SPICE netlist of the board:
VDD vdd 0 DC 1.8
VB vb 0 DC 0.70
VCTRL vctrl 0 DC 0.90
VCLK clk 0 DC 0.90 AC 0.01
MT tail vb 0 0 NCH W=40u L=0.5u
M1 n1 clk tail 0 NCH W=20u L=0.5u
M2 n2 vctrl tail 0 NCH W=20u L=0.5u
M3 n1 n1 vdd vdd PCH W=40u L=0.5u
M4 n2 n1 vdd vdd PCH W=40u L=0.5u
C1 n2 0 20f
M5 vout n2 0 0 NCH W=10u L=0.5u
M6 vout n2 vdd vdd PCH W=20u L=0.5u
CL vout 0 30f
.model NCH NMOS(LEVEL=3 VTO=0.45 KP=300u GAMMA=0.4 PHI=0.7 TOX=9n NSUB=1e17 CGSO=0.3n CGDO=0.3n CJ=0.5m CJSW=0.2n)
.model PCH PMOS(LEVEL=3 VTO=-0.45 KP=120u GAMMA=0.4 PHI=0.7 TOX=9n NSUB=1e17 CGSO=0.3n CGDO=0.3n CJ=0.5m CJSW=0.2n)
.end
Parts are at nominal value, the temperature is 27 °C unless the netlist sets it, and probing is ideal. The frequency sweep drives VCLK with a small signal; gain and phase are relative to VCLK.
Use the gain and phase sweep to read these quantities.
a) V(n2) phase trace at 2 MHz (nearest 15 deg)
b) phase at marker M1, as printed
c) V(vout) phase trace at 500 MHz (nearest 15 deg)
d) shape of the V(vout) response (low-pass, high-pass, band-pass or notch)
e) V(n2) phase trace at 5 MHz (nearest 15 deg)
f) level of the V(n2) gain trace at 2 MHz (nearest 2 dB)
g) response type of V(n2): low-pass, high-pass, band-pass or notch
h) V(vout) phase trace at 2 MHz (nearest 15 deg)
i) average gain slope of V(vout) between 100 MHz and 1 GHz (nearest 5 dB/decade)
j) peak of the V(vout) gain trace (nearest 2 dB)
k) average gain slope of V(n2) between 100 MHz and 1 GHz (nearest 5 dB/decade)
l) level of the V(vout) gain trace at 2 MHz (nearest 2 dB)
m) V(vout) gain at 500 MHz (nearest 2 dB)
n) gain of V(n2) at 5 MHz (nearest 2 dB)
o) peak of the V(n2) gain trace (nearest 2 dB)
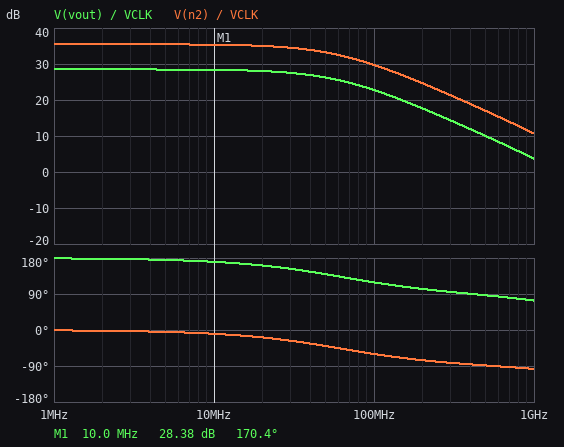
0 deg
170.4 deg
90 deg
low-pass
0 deg
36 dB
low-pass
180 deg
-20 dB/decade
28 dB
-20 dB/decade
28 dB
10 dB
36 dB
36 dB
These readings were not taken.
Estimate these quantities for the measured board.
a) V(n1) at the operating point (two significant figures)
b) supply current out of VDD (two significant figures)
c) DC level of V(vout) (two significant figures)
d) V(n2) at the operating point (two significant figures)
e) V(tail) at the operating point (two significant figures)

1.1 V
820 µA
47 mV
1.1 V
180 mV
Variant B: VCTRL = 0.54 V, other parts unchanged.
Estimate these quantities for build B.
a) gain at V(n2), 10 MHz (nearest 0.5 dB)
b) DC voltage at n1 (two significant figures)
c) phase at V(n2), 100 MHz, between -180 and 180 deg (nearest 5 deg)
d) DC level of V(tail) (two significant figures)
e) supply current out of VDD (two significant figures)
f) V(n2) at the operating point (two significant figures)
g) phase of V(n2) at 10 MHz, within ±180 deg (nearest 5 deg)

-67.5 dB
1.0 V
-95 deg
120 mV
530 µA
1.8 V
-90 deg
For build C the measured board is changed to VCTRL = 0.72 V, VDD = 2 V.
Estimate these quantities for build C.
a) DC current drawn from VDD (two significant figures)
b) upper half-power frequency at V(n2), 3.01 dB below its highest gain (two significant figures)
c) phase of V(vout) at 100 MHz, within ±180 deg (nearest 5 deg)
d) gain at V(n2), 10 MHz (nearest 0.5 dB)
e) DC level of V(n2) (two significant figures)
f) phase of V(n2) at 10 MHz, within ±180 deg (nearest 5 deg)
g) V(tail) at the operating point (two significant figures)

560 µA
2.0 GHz
85 deg
-11.0 dB
2.0 V
0 deg
130 mV
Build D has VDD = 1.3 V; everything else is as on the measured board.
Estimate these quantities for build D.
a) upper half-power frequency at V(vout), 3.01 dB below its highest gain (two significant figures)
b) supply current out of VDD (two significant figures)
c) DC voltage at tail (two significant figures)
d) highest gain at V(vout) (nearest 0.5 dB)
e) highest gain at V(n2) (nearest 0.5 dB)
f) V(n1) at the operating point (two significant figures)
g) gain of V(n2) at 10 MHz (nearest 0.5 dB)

65 MHz
700 µA
170 mV
33.5 dB
33.0 dB
590 mV
32.5 dB
